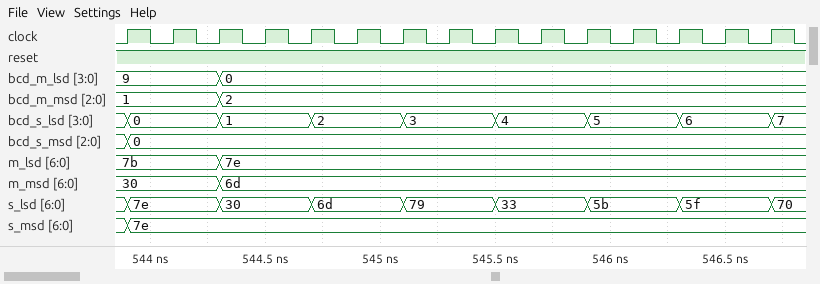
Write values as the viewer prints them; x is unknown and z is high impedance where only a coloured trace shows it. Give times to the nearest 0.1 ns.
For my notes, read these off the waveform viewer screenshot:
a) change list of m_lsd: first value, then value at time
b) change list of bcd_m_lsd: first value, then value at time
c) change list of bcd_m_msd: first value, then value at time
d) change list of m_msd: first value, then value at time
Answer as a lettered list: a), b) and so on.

a) 7b, 7e at 544.3 ns
b) 9, 0 at 544.3 ns
c) 1, 2 at 544.3 ns
d) 30, 6d at 544.3 ns
